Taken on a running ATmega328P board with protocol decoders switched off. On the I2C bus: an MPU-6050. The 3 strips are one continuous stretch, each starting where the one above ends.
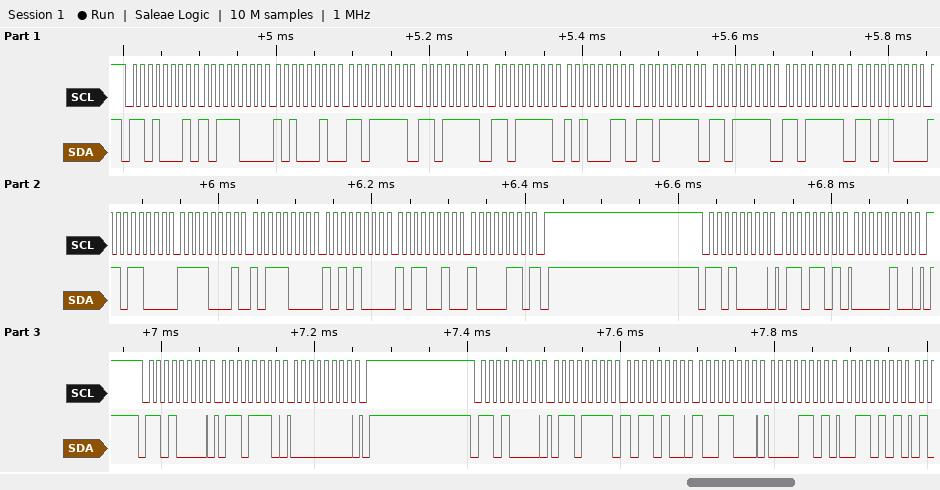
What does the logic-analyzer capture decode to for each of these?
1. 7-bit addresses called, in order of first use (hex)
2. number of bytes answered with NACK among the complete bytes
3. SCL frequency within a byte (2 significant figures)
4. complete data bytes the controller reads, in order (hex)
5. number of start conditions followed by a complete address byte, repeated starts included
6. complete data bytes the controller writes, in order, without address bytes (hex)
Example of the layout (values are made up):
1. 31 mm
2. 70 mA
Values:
1. 0x68
2. 1
3. 100 kHz
4. B8 A2 DF DF DF A3 DF DF DF D8 D8 F1 B8 A8 B2 86
5. 4
6. 6D 04 6E 00 6F B4 98 0D 35
